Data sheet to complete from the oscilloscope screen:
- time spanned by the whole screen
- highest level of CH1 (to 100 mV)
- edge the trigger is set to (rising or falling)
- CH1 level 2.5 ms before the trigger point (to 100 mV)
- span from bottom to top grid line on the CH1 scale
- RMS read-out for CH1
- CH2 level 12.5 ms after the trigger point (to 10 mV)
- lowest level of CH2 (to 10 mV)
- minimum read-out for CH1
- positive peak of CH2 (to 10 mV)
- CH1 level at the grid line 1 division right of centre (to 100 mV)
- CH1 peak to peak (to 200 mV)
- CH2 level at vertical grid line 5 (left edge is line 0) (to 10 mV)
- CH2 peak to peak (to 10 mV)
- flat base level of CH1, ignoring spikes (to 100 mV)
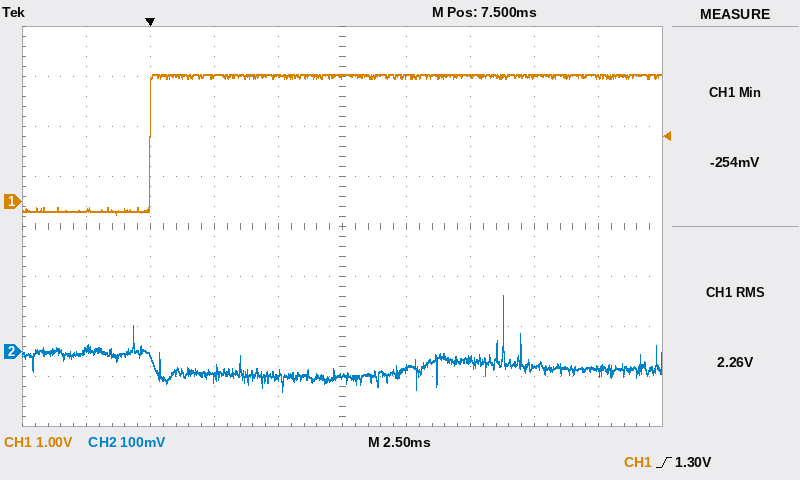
25 ms
2.5 V
rising
-200 mV
8 V
2.26 V
-20 mV
-80 mV
-254 mV
110 mV
2.5 V
2.8 V
-50 mV
190 mV
-200 mV
